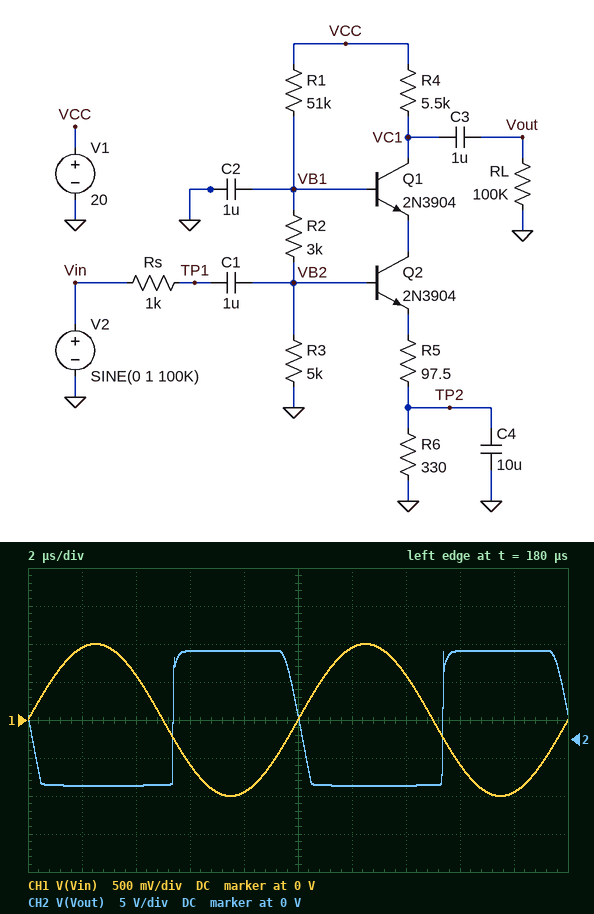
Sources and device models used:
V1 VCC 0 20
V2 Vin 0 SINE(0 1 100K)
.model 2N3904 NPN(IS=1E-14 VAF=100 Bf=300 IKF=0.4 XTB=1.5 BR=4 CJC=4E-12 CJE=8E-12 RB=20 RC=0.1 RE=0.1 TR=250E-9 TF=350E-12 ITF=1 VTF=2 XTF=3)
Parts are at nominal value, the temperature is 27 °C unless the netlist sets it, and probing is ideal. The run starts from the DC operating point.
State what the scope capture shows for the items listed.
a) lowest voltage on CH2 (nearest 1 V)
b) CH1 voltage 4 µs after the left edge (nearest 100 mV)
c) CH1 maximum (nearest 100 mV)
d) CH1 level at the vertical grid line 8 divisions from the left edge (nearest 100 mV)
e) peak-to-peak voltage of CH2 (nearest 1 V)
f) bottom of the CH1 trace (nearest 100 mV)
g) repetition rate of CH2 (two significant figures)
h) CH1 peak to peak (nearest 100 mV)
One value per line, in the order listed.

-6 V
600 mV
1.0 V
-600 mV
18 V
-1.0 V
100 kHz
2.0 V
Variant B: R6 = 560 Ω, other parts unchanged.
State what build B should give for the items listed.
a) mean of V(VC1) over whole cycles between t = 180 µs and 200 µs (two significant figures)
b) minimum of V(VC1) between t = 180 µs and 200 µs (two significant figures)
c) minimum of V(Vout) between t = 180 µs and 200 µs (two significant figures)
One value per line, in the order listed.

11 V
1.7 V
-10 V
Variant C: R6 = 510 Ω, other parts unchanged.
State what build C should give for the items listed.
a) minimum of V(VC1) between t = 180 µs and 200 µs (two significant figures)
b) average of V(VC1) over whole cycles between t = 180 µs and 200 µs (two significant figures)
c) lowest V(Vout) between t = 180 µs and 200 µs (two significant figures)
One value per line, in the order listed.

1.7 V
11 V
-9.5 V
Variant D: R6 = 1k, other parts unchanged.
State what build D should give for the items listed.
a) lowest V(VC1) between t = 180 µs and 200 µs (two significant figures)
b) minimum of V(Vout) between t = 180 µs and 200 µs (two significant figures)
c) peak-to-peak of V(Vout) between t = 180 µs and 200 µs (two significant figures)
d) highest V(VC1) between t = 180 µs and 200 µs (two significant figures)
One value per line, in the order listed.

1.8 V
-13 V
18 V
20 V
